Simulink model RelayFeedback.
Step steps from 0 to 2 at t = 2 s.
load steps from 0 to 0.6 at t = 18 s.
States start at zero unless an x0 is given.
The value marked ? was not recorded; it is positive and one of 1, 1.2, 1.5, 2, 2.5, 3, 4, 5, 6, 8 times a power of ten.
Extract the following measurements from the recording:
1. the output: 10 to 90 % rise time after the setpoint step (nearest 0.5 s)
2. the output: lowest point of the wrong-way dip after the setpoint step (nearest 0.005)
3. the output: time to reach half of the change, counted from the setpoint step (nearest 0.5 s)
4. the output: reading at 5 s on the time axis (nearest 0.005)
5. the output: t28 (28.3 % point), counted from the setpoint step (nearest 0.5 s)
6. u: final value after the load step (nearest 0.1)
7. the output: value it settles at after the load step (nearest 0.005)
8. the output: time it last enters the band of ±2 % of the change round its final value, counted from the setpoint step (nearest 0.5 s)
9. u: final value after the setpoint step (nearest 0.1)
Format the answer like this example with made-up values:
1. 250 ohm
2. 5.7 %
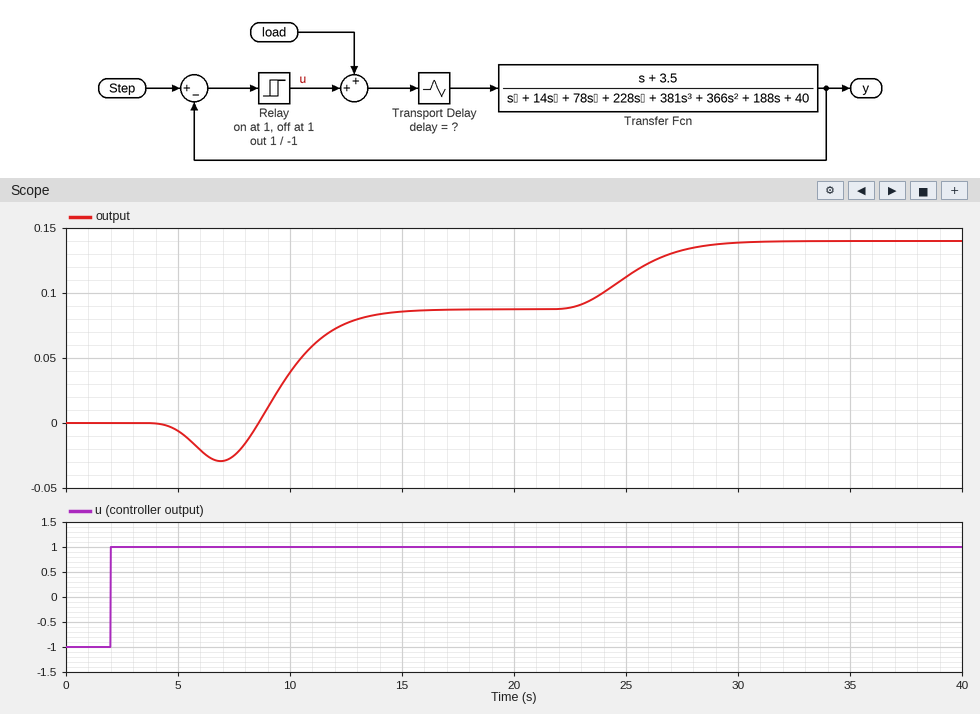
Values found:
1. 4.0 s
2. -0.030
3. 8.0 s
4. -0.005
5. 7.5 s
6. 1.0
7. 0.140
8. 13.0 s
9. 1.0
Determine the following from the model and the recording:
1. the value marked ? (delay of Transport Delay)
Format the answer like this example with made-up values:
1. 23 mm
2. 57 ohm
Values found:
1. 3
